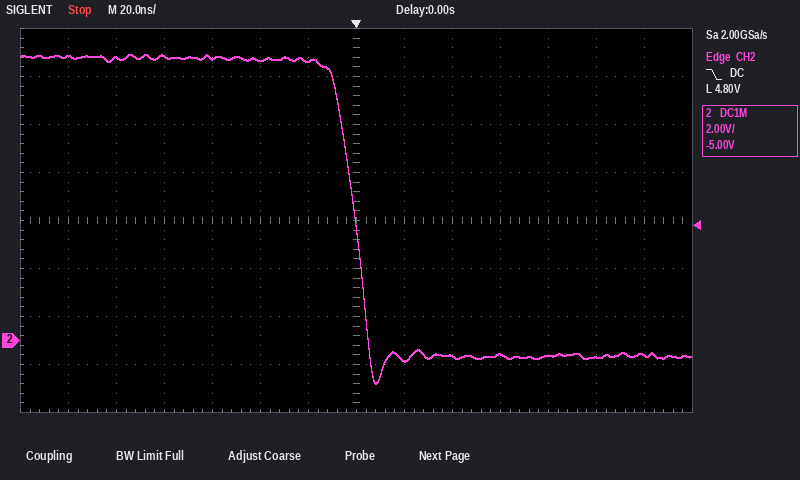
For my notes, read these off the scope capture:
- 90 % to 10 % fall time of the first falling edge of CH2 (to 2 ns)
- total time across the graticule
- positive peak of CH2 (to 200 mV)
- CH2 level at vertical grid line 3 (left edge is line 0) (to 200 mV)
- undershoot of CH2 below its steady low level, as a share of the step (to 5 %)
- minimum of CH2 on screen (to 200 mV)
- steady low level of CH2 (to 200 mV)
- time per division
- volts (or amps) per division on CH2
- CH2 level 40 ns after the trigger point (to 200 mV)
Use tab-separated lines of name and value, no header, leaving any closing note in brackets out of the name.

90 % to 10 % fall time of the first falling edge of CH2	14 ns
total time across the graticule	280 ns
positive peak of CH2	12.0 V
CH2 level at vertical grid line 3 (left edge is line 0)	11.8 V
undershoot of CH2 below its steady low level, as a share of the step	10 %
minimum of CH2 on screen	-1.8 V
steady low level of CH2	-600 mV
time per division	20 ns
volts (or amps) per division on CH2	2 V
CH2 level 40 ns after the trigger point	-600 mV
